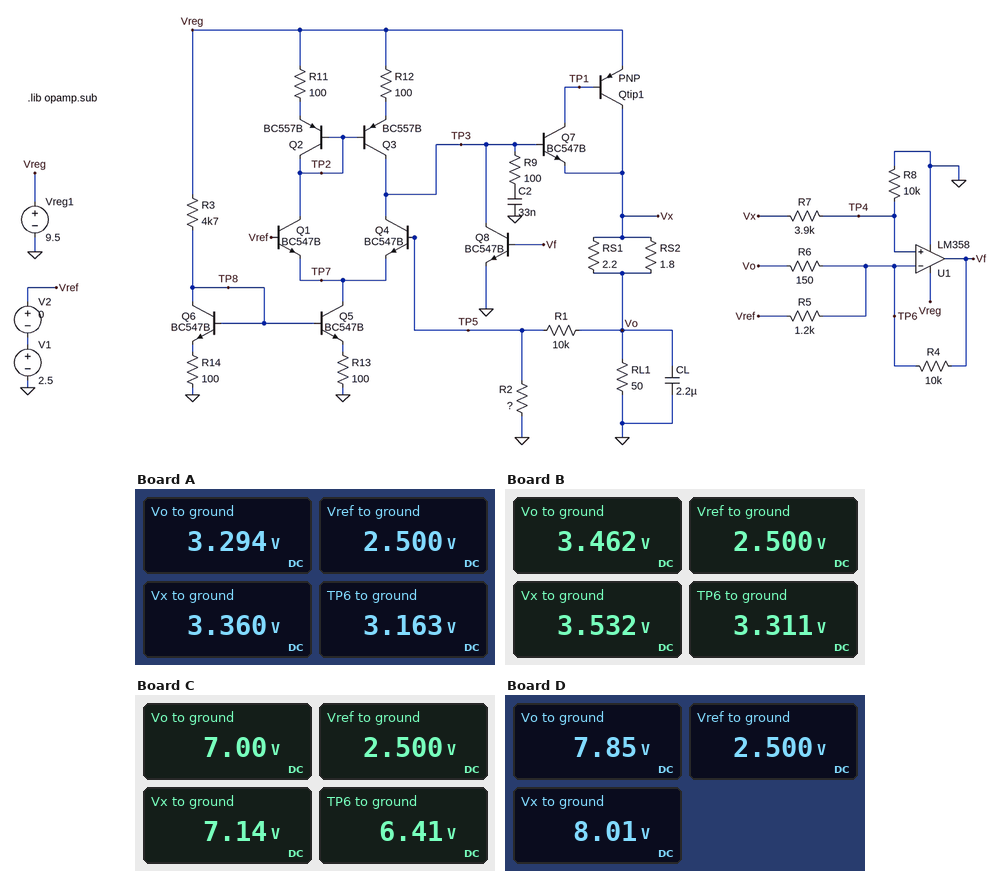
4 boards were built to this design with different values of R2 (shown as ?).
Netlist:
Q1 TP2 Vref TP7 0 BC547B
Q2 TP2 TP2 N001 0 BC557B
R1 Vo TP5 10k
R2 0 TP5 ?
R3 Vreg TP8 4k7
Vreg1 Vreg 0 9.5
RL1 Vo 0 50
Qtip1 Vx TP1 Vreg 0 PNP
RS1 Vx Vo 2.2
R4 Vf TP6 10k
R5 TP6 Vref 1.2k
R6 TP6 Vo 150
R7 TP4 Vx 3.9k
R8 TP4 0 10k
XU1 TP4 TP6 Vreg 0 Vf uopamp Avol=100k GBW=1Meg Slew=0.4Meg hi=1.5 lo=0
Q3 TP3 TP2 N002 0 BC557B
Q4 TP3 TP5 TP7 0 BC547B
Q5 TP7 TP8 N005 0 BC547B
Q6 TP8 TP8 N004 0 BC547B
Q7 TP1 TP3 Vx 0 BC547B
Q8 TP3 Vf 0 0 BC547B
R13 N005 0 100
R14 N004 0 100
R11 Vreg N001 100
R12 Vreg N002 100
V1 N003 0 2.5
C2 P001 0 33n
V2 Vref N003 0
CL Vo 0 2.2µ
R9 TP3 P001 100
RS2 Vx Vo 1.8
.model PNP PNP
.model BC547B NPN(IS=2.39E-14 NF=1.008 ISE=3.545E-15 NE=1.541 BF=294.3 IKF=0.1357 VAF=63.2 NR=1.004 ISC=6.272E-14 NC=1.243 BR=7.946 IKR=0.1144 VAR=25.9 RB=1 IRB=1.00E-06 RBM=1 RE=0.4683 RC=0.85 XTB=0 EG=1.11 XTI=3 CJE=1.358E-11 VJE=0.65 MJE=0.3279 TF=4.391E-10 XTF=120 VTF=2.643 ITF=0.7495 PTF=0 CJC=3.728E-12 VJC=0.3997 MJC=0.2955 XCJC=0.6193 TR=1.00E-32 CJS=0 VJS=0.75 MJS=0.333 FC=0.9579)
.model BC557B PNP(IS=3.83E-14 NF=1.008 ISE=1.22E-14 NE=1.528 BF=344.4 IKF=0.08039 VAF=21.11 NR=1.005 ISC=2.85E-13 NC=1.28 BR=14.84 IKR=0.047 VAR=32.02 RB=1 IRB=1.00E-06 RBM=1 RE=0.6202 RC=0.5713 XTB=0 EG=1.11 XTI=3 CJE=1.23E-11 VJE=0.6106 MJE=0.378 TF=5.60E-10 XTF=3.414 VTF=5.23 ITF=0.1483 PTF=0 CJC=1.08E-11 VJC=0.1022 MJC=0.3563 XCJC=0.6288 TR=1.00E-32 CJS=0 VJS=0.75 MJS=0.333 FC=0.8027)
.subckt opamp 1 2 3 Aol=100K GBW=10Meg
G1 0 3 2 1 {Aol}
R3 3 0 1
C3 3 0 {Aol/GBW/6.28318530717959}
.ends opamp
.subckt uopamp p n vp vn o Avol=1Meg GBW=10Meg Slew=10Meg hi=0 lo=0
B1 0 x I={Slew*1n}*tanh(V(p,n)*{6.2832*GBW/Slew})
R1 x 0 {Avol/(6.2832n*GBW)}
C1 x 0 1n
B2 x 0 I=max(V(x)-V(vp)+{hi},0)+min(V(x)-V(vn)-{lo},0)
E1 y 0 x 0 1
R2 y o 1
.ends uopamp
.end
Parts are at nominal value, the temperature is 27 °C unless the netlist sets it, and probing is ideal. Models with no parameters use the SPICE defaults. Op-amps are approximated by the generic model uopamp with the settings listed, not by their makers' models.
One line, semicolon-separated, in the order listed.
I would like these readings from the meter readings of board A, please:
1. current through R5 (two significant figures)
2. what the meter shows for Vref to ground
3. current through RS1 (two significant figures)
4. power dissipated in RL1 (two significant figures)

550 µA; 2.500 V; 30 mA; 220 mW
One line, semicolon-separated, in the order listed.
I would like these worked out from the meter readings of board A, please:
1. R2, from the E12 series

33 kΩ
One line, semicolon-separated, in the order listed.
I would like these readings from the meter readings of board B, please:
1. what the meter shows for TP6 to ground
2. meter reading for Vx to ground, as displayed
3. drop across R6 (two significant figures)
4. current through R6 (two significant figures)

3.311 V; 3.532 V; 150 mV; 1.0 mA
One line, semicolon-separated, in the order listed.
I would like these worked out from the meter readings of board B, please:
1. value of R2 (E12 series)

27 kΩ
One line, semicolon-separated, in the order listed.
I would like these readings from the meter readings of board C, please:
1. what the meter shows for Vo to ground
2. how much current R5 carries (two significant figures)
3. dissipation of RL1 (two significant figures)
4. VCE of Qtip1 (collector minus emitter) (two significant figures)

7.00 V; 3.3 mA; 980 mW; -2.4 V
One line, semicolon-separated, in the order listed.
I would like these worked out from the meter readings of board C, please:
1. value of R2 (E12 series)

5.6 kΩ
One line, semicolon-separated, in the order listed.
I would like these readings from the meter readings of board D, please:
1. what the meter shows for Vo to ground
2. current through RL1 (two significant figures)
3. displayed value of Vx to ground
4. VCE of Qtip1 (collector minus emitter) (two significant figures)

7.85 V; 160 mA; 8.01 V; -1.5 V
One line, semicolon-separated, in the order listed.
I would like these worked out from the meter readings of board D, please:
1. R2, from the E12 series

4.7 kΩ
